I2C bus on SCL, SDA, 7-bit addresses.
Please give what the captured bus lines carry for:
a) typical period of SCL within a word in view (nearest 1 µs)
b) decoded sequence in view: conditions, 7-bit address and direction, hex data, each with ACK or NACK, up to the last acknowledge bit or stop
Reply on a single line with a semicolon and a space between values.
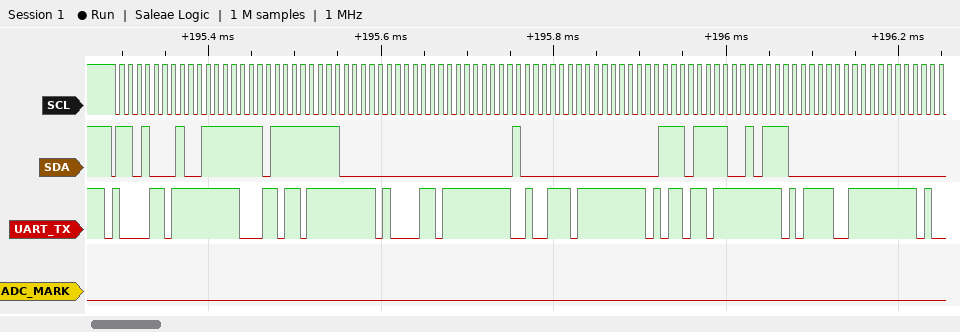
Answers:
10 µs; start, address 68 read ACK, 7F ACK, FF ACK, 00 ACK, 00 ACK, 40 ACK, 00 ACK, EF ACK, 5C ACK, 00 ACK
